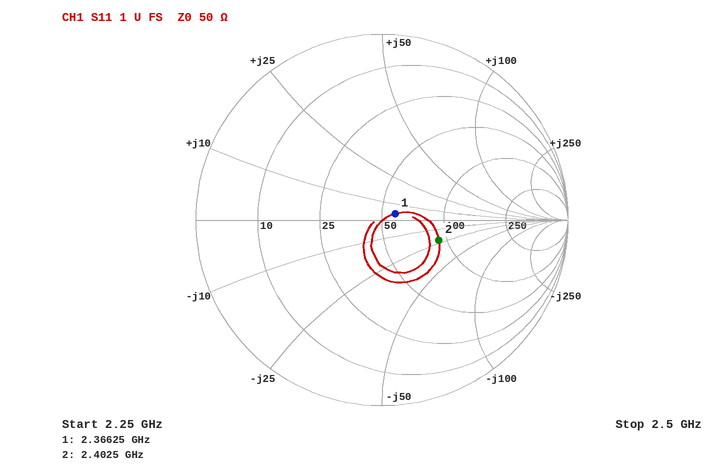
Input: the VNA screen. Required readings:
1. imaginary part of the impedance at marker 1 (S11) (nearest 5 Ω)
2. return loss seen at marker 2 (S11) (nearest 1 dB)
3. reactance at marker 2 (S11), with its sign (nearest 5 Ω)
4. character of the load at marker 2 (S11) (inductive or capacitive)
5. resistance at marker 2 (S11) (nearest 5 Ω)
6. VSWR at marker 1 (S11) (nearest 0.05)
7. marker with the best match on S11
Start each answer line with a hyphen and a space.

- +5 Ω
- 10 dB
- -20 Ω
- capacitive
- 90 Ω
- 1.15
- marker 1
